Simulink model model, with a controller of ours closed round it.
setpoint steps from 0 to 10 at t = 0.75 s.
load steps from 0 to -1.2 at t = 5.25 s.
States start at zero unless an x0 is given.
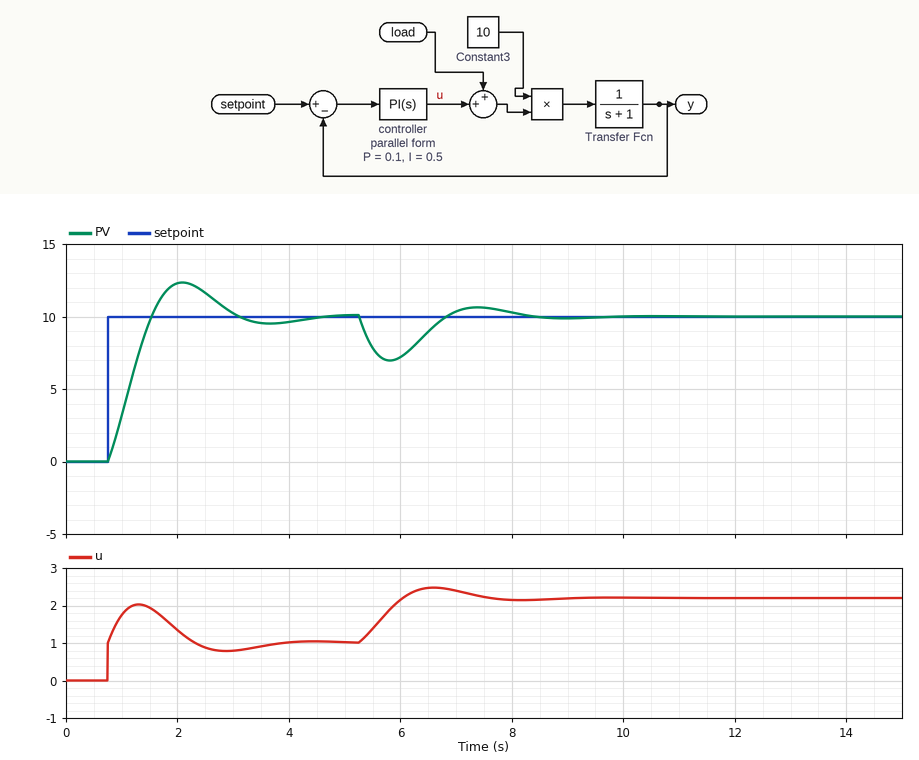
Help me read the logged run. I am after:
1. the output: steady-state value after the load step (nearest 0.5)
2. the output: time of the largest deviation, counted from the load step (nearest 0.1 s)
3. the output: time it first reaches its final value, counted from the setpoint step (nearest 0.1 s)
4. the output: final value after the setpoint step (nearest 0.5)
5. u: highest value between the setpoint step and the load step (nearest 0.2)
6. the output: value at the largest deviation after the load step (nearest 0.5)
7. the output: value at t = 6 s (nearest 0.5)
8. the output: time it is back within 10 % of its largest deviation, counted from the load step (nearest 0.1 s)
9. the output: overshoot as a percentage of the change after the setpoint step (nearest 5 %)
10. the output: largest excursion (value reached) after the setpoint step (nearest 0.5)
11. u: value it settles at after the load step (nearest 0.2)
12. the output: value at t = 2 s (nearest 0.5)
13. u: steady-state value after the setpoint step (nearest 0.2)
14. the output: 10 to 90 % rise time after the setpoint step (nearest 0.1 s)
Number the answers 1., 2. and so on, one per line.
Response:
1. 10.0
2. 0.6 s
3. 0.8 s
4. 10.0
5. 2.0
6. 7.0
7. 7.0
8. 2.7 s
9. 25 %
10. 12.5
11. 2.2
12. 12.5
13. 1.0
14. 0.6 s
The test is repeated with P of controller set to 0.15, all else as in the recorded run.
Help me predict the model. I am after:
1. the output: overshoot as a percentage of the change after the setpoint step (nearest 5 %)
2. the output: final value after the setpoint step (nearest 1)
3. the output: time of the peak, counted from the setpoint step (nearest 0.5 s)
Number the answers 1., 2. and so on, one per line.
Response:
1. 15 %
2. 10
3. 1.5 s
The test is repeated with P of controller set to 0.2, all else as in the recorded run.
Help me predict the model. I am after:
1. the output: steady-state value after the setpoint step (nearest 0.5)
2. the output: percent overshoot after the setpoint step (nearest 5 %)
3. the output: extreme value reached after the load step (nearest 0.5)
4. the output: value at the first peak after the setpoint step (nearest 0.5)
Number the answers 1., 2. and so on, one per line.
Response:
1. 10.0
2. 10 %
3. 7.5
4. 11.0
